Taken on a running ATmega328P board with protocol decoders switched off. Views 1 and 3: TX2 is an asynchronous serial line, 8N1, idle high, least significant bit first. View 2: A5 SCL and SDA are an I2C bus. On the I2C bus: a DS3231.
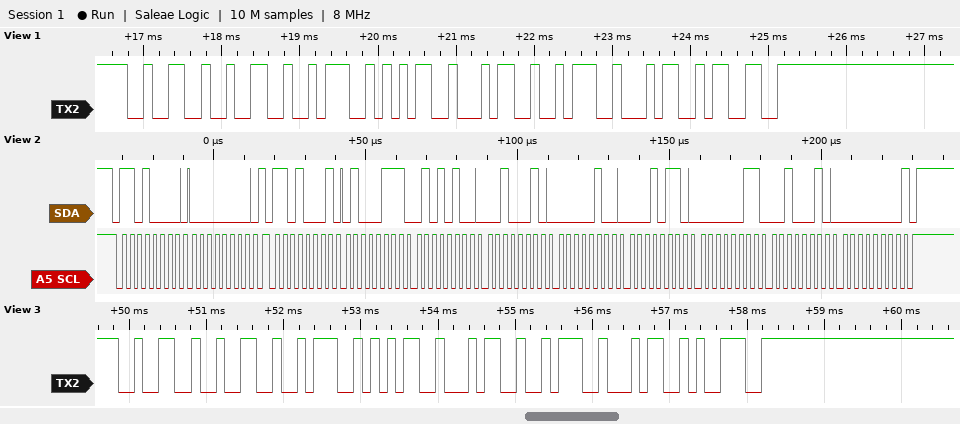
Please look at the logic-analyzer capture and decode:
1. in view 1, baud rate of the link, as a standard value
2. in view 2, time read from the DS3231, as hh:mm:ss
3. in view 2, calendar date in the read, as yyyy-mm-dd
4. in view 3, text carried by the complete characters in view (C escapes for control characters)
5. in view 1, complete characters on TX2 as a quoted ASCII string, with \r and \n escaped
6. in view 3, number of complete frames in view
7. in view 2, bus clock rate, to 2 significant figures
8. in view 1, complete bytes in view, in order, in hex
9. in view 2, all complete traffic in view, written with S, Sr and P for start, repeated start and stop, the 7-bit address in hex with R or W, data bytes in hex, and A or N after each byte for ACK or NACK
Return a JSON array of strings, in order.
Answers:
["9600 baud", "22:54:47", "2022-03-16", "\"22:54:49\"", "\"22:54:43\"", "8", "400 kHz", "0x32 0x32 0x3A 0x35 0x34 0x3A 0x34 0x33", "S 68W A 00 A Sr 68R A 47 A 54 A 22 A 04 A 16 A 03 A 22 A 00 N P"]
